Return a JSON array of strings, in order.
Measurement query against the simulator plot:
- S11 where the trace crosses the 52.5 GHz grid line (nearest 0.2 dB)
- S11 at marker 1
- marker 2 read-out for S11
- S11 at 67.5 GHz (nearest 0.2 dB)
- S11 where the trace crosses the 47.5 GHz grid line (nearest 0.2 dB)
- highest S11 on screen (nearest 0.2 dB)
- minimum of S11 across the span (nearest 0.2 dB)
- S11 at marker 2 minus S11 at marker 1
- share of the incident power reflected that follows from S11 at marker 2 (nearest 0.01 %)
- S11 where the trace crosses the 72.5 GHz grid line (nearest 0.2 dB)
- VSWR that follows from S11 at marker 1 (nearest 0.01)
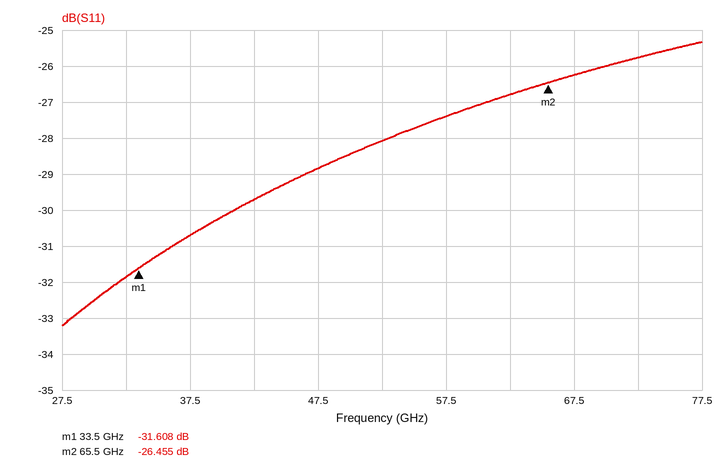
["-28.0 dB", "-31.608 dB", "-26.455 dB", "-26.2 dB", "-28.8 dB", "-25.4 dB", "-33.2 dB", "5.153 dB", "0.23 %", "-25.8 dB", "1.05"]
